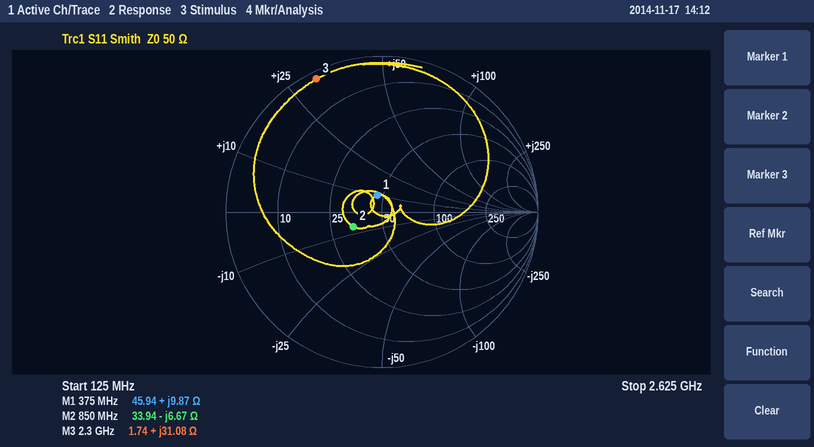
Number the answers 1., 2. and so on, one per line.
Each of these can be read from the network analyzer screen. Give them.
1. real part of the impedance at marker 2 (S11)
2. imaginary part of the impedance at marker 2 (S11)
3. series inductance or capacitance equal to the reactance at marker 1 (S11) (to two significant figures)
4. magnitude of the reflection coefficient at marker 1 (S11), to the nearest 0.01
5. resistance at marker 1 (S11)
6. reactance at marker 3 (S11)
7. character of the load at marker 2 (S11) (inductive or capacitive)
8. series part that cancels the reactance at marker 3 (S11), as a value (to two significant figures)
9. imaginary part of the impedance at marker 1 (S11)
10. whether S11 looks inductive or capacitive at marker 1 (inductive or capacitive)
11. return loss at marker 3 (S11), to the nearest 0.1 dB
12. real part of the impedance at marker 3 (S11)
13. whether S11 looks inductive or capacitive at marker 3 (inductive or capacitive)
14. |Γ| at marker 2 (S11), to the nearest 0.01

1. 33.94 Ω
2. -6.67 Ω
3. 4.2 nH
4. 0.11
5. 45.94 Ω
6. +31.08 Ω
7. capacitive
8. 2.2 pF
9. +9.87 Ω
10. inductive
11. 0.4 dB
12. 1.74 Ω
13. inductive
14. 0.21
